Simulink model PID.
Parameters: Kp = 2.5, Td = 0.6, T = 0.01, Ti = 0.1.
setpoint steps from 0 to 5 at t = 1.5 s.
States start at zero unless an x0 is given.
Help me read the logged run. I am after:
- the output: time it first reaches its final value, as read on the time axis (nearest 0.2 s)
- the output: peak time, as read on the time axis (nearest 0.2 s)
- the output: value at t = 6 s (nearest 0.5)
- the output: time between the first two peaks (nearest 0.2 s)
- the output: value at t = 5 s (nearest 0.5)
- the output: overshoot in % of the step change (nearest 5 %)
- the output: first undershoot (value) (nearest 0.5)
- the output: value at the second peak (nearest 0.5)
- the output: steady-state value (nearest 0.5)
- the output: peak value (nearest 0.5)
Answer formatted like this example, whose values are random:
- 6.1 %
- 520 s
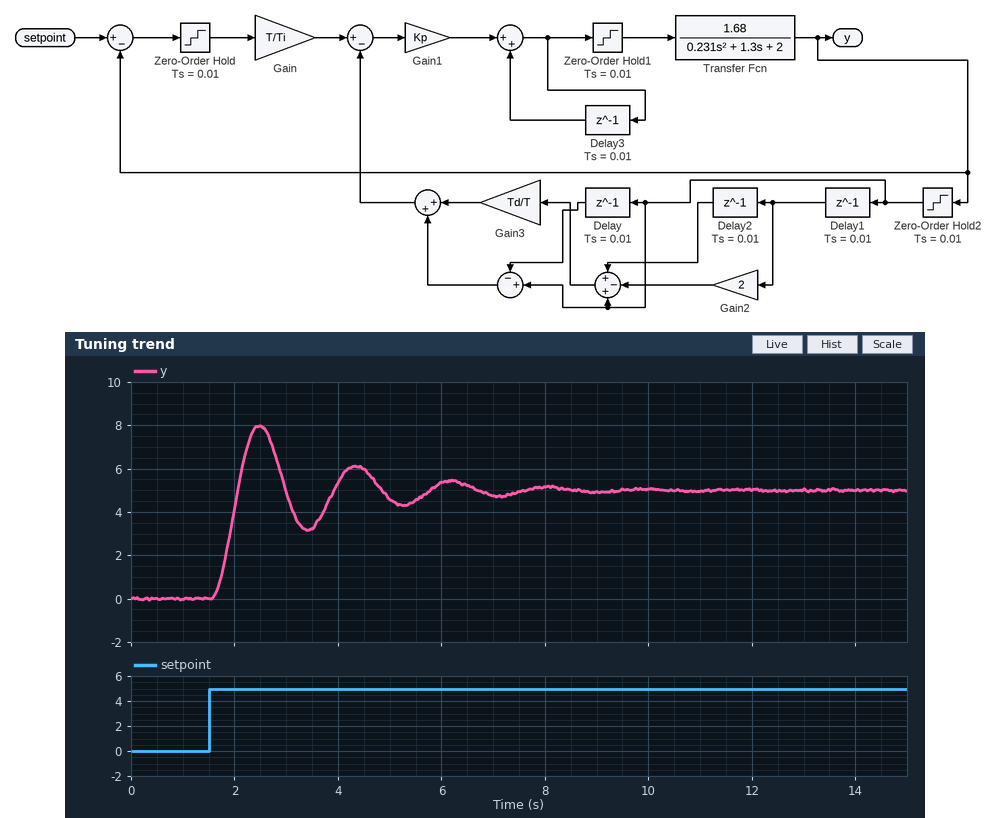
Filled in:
- 2.0 s
- 2.4 s
- 5.5
- 1.8 s
- 4.5
- 60 %
- 3.0
- 6.0
- 5.0
- 8.0
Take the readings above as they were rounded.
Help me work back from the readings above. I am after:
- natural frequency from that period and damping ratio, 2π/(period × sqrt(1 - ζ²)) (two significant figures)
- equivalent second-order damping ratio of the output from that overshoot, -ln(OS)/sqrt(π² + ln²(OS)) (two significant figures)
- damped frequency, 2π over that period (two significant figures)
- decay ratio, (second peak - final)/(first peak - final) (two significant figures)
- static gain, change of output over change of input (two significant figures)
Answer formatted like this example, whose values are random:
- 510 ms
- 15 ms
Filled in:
- 3.5 rad/s
- 0.16
- 3.5 rad/s
- 0.33
- 1.0
